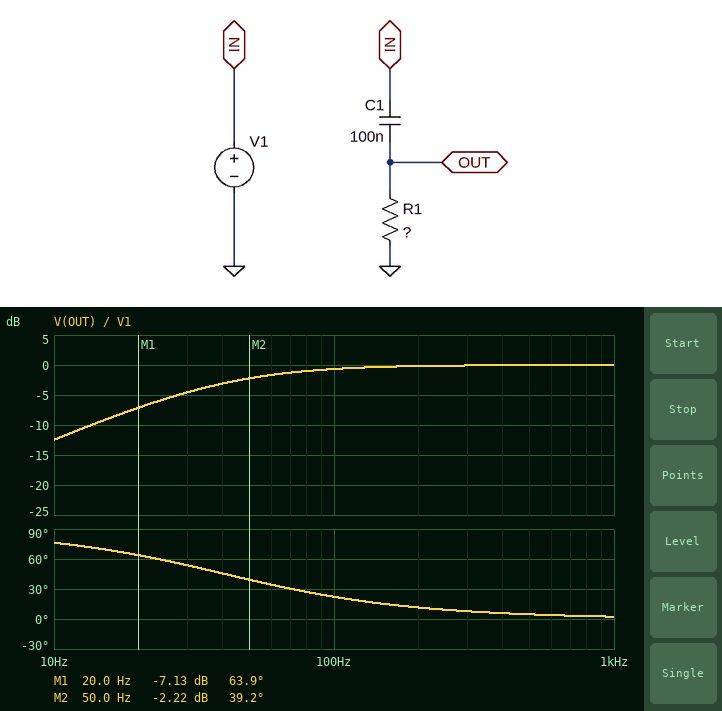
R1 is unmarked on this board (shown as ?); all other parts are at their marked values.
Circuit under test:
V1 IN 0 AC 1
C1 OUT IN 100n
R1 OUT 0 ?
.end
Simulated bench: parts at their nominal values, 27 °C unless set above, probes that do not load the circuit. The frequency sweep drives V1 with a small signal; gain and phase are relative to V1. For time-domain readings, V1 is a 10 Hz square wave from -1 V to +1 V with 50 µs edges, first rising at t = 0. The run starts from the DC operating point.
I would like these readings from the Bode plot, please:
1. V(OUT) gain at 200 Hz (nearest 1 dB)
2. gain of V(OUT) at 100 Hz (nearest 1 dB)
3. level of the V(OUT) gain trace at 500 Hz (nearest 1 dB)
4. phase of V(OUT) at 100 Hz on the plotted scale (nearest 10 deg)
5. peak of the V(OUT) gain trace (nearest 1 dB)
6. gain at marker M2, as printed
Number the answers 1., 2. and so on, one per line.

1. 0 dB
2. -1 dB
3. 0 dB
4. 20 deg
5. 0 dB
6. -2.22 dB
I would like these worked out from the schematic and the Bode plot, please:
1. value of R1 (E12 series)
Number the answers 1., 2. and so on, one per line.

1. 39 kΩ
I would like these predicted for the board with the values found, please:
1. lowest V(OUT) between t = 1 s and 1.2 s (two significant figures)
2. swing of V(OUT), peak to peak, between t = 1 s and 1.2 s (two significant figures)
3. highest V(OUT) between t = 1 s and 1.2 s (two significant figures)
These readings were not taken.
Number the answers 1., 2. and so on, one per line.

1. -2.0 V
2. 4.0 V
3. 2.0 V
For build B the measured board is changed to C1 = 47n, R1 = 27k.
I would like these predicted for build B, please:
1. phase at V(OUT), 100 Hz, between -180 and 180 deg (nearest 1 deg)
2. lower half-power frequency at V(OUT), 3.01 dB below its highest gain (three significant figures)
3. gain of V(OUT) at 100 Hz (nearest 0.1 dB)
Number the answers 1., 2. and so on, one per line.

1. 51 deg
2. 125 Hz
3. -4.1 dB
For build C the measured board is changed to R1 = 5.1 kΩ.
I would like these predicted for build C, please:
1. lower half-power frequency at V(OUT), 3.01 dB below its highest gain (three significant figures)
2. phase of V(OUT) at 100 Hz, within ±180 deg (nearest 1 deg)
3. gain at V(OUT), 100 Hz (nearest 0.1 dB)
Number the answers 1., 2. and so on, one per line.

1. 312 Hz
2. 72 deg
3. -10.3 dB
